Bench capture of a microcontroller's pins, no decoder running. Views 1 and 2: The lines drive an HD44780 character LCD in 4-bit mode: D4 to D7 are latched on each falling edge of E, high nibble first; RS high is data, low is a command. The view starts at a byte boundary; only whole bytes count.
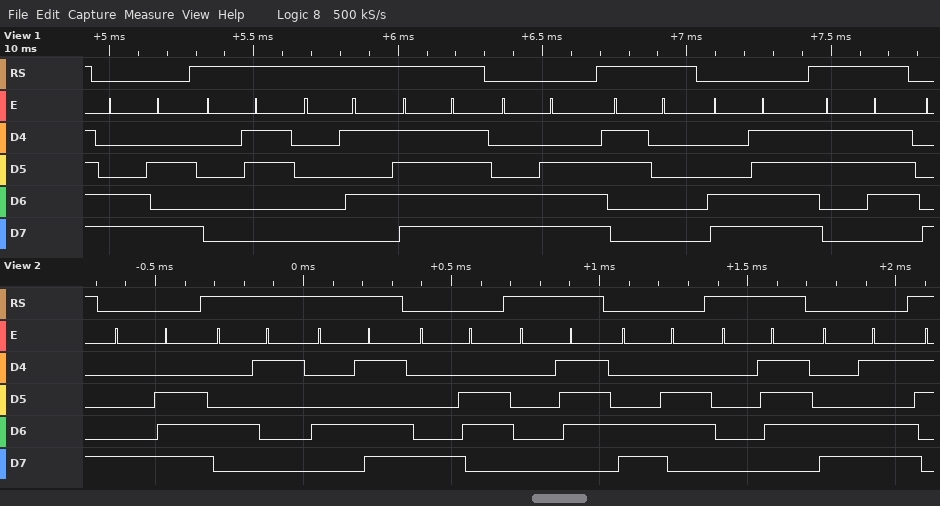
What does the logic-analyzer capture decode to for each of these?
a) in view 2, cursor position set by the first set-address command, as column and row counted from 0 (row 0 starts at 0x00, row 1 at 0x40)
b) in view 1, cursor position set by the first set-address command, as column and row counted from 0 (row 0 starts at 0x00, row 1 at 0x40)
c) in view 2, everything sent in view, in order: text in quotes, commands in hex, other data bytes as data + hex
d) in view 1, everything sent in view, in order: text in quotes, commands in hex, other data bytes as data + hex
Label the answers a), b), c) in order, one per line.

a) column 14, row 0
b) column 10, row 1
c) 0x8E "AM" 0x86 data 07 0xC6 data 07 0xCD
d) 0xCA data 03 05 FF 0xCE "0" 0xCF "7"
